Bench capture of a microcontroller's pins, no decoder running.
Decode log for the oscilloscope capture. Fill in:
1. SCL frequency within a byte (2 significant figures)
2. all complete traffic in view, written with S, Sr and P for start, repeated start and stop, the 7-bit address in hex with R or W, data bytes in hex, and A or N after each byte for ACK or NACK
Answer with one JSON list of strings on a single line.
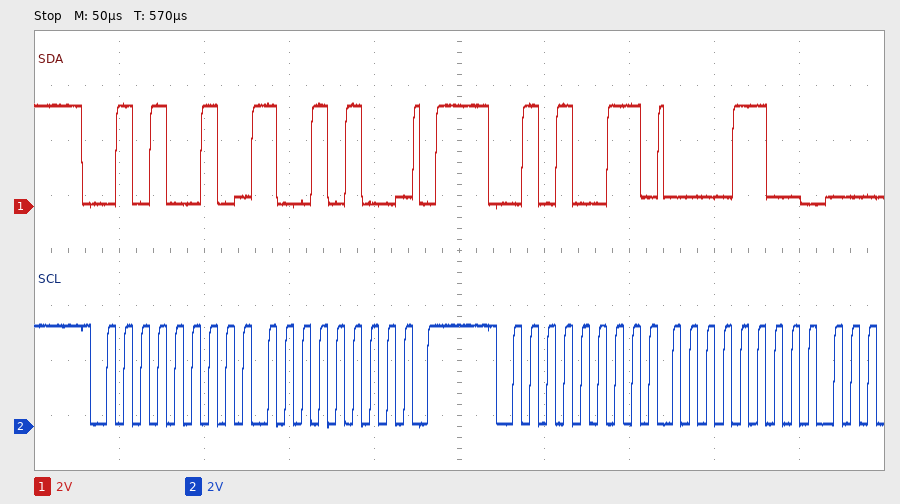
["100 kHz", "S 29W A 94 A P S 29R A 0C A"]
